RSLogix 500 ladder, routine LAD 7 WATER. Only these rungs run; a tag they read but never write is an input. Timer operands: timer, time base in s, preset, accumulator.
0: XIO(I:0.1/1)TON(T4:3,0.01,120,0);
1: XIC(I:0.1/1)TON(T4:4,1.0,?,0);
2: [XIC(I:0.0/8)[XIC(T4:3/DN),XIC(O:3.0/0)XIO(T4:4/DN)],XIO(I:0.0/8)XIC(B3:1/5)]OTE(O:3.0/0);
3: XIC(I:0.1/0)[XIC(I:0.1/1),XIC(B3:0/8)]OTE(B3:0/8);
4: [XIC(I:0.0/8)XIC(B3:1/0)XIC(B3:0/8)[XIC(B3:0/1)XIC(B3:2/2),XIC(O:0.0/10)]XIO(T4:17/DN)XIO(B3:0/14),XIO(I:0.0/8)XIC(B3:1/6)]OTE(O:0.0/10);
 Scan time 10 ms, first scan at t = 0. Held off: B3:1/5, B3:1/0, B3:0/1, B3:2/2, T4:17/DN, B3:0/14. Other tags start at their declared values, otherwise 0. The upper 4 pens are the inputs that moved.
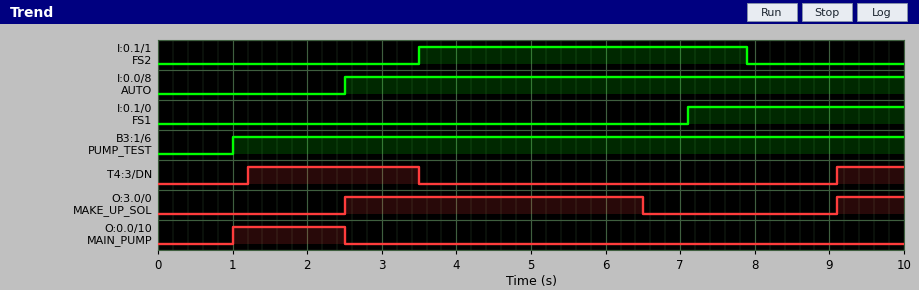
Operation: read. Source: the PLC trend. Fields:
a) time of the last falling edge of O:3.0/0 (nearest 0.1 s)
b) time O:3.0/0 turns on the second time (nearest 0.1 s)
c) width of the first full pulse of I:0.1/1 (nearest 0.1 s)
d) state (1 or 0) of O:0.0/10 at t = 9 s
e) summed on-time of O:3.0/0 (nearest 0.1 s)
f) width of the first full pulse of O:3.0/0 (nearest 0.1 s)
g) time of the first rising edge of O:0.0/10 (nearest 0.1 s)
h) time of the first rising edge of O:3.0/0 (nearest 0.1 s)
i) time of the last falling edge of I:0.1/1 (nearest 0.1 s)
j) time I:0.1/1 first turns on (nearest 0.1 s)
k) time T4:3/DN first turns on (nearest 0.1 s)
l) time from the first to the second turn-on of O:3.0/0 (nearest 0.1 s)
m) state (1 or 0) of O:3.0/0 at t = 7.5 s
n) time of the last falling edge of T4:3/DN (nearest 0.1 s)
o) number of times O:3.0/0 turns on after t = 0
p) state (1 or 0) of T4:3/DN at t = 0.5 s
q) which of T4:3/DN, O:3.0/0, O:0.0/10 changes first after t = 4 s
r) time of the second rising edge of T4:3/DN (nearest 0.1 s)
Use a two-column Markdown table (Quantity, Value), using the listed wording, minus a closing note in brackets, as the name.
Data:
| Quantity | Value |
|---|---|
| time of the last falling edge of O:3.0/0 | 6.5 s |
| time O:3.0/0 turns on the second time | 9.1 s |
| width of the first full pulse of I:0.1/1 | 4.4 s |
| state (1 or 0) of O:0.0/10 at t = 9 s | 0 |
| summed on-time of O:3.0/0 | 4.9 s |
| width of the first full pulse of O:3.0/0 | 4.0 s |
| time of the first rising edge of O:0.0/10 | 1.0 s |
| time of the first rising edge of O:3.0/0 | 2.5 s |
| time of the last falling edge of I:0.1/1 | 7.9 s |
| time I:0.1/1 first turns on | 3.5 s |
| time T4:3/DN first turns on | 1.2 s |
| time from the first to the second turn-on of O:3.0/0 | 6.6 s |
| state (1 or 0) of O:3.0/0 at t = 7.5 s | 0 |
| time of the last falling edge of T4:3/DN | 3.5 s |
| number of times O:3.0/0 turns on after t = 0 | 2 |
| state (1 or 0) of T4:3/DN at t = 0.5 s | 0 |
| which of T4:3/DN, O:3.0/0, O:0.0/10 changes first after t = 4 s | O:3.0/0 |
| time of the second rising edge of T4:3/DN | 9.1 s |
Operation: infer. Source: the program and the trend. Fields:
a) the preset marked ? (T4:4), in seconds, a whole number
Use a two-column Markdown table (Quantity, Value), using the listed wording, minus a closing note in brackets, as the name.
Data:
| Quantity | Value |
|---|---|
| the preset marked ? (T4:4), in seconds, a whole number | 3 s |
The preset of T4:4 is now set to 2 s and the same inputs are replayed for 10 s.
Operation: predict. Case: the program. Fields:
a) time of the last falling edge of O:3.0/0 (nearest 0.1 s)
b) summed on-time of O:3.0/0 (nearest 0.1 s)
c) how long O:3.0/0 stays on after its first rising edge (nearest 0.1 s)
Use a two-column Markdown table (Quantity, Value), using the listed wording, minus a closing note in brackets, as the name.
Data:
| Quantity | Value |
|---|---|
| time of the last falling edge of O:3.0/0 | 5.5 s |
| summed on-time of O:3.0/0 | 3.9 s |
| how long O:3.0/0 stays on after its first rising edge | 3.0 s |
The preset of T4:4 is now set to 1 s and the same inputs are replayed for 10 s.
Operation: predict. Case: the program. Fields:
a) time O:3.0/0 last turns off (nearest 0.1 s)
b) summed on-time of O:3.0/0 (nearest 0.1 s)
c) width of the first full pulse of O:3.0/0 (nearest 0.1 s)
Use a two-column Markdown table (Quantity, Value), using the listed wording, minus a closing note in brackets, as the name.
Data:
| Quantity | Value |
|---|---|
| time O:3.0/0 last turns off | 4.5 s |
| summed on-time of O:3.0/0 | 2.9 s |
| width of the first full pulse of O:3.0/0 | 2.0 s |
